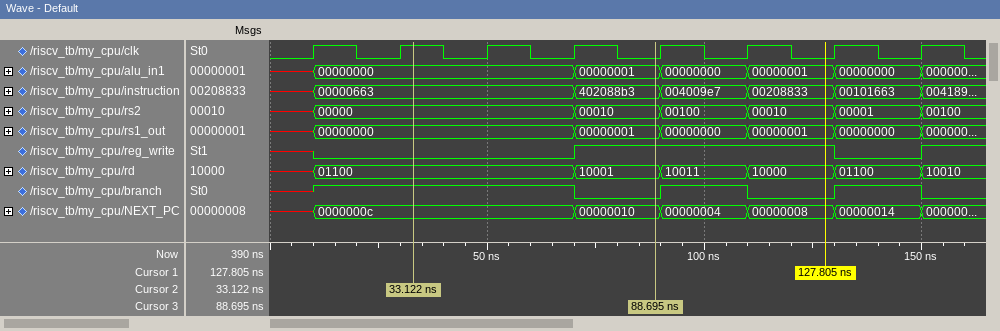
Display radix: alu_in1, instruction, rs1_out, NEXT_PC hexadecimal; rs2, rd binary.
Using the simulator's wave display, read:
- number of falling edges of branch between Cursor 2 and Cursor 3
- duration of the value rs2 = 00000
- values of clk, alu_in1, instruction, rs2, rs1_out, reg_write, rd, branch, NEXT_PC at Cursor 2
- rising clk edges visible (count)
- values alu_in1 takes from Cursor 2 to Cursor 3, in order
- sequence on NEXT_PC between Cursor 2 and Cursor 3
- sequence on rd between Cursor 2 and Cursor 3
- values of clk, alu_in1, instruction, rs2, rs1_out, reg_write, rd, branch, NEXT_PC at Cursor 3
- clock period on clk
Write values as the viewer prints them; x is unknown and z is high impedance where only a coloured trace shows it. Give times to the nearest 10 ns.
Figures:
1
60 ns
clk=1, alu_in1=00000000, instruction=00000663, rs2=00000, rs1_out=00000000, reg_write=0, rd=01100, branch=1, NEXT_PC=0000000c
8
00000000, 00000001
0000000c, 00000010
01100, 10001
clk=0, alu_in1=00000001, instruction=402088b3, rs2=00010, rs1_out=00000001, reg_write=1, rd=10001, branch=0, NEXT_PC=00000010
20 ns
